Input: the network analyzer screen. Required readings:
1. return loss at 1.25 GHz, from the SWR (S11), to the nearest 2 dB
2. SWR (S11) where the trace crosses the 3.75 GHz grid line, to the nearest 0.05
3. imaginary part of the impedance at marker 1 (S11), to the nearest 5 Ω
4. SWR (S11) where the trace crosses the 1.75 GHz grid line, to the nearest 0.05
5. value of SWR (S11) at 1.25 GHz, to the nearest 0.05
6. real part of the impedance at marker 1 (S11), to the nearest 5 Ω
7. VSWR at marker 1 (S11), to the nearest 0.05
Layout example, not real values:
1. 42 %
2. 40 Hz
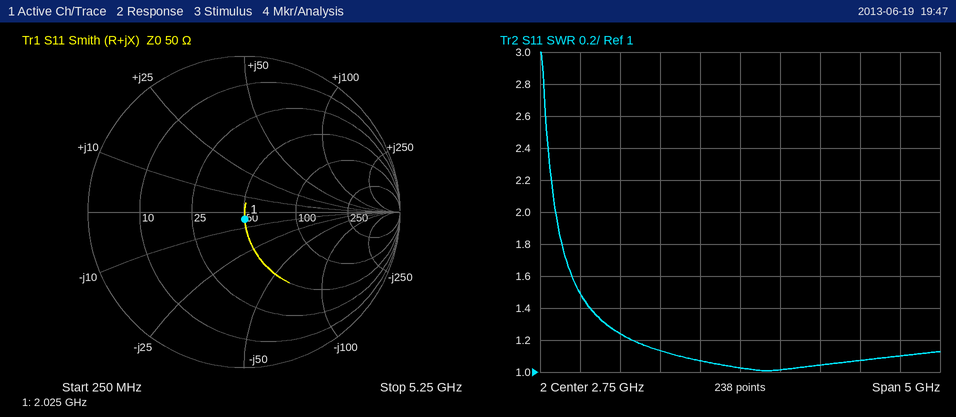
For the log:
1. 20 dB
2. 1.05
3. -5 Ω
4. 1.15
5. 1.25
6. 50 Ω
7. 1.10
